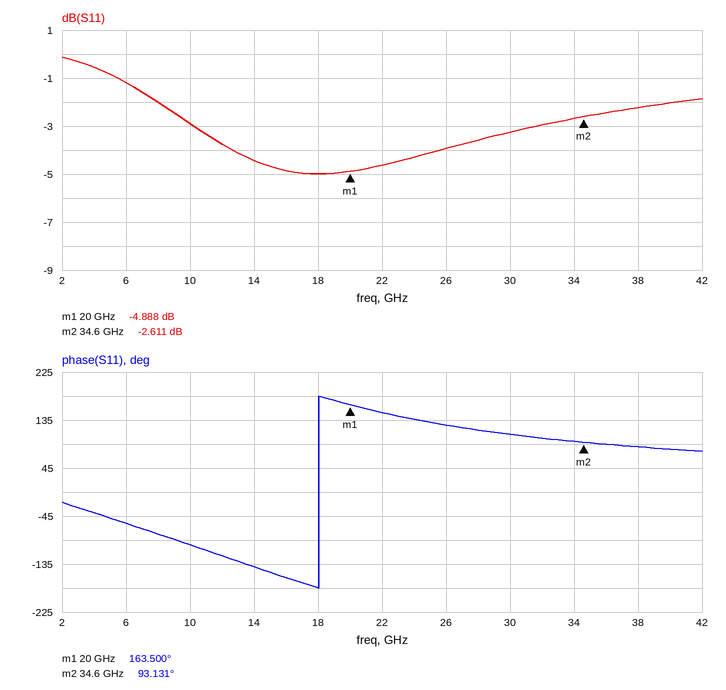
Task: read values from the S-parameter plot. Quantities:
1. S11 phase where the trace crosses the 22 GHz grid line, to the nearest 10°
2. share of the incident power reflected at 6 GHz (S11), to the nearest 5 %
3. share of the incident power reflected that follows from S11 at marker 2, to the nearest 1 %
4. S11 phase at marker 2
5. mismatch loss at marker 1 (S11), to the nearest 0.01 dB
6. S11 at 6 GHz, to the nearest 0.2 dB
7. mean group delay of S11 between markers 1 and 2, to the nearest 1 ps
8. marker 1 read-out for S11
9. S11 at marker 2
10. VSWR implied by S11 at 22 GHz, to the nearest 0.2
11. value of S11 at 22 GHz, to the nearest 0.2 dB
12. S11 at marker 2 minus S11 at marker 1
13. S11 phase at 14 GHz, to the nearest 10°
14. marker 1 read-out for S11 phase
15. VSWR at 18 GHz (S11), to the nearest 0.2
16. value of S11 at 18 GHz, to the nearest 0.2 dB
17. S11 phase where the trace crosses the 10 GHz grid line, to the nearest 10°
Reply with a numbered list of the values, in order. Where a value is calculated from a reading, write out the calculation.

1. 150°
2. 10^(-1.2/10) ≈ 75.9 %, so 75 % to the nearest 5 %
3. 10^(-2.611/10) ≈ 55 %
4. 93.131°
5. −10 log10(1 − 10^(-4.888/10)) ≈ 1.70 dB
6. -1.2 dB
7. −(93.131° − (163.5°))/(360° × 14.6 GHz) ≈ 13 ps
8. -4.888 dB
9. -2.611 dB
10. |Γ| = 10^(-4.6/20) = 0.5888; VSWR = (1 + 0.5888)/(1 − 0.5888) ≈ 3.86, so 3.8 to the nearest 0.2
11. -4.6 dB
12. -2.611 − (-4.888) = 2.277 dB
13. -140°
14. 163.500°
15. |Γ| = 10^(-5/20) = 0.5623; VSWR = (1 + 0.5623)/(1 − 0.5623) ≈ 3.6
16. -5.0 dB
17. -100°
